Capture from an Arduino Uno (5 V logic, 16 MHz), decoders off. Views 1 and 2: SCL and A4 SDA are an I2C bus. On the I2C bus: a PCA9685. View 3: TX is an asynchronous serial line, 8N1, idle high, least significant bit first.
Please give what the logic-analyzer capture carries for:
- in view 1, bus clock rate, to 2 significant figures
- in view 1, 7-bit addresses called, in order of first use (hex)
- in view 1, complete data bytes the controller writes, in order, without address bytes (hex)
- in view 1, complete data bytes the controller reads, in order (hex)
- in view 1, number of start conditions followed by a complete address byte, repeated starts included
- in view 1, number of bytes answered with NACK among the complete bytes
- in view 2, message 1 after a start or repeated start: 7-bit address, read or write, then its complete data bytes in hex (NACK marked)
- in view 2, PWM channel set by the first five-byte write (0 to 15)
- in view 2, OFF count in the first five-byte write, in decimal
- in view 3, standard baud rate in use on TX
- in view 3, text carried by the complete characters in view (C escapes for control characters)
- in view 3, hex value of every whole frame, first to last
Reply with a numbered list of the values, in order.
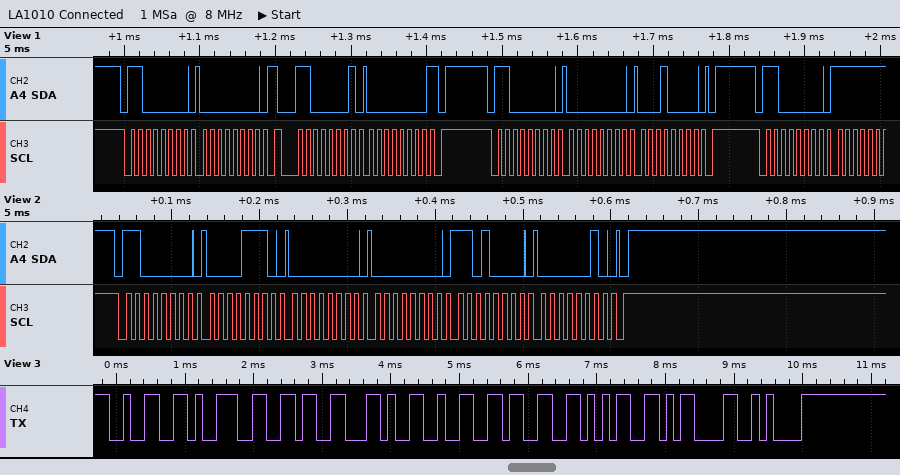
1. 100 kHz
2. 0x60
3. 00 00 10
4. 00
5. 4
6. 1
7. 0x60 write: 0E 00 00 D0 02
8. 2
9. 720
10. 9600 baud
11. "296,235\r\n"
12. 32 39 36 2C 32 33 35 0D 0A
